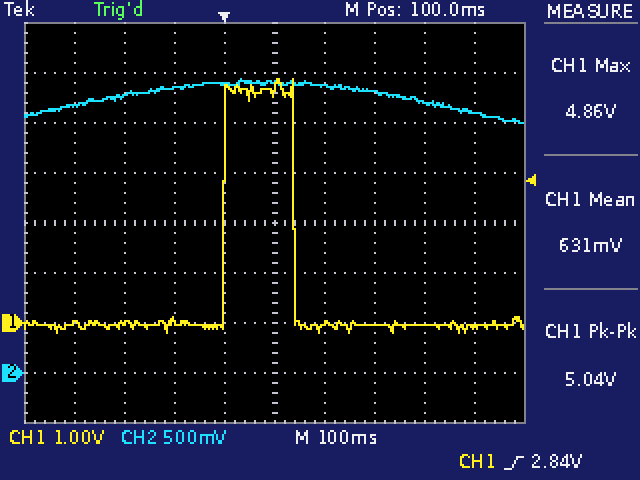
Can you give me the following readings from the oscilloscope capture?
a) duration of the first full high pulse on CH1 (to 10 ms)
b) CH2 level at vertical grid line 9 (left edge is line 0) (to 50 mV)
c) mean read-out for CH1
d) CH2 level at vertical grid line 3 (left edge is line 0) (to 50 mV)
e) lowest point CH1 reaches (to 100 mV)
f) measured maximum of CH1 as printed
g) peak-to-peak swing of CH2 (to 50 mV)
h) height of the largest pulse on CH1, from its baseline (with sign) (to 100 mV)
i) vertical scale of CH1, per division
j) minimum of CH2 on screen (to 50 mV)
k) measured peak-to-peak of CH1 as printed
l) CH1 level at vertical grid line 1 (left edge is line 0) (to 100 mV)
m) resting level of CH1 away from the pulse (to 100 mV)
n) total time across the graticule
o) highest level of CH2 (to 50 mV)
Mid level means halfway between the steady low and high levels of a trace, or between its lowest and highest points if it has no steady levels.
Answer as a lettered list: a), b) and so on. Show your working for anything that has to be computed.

a) 140 ms
b) 2.60 V
c) 631 mV
d) 2.85 V
e) -200 mV
f) 4.86 V
g) 2.95 V − (2.50 V) = 450 mV
h) +4.9 V
i) 1 V
j) 2.50 V
k) 5.04 V
l) 0.0 V
m) 0.0 V
n) 1 s
o) 2.95 V
